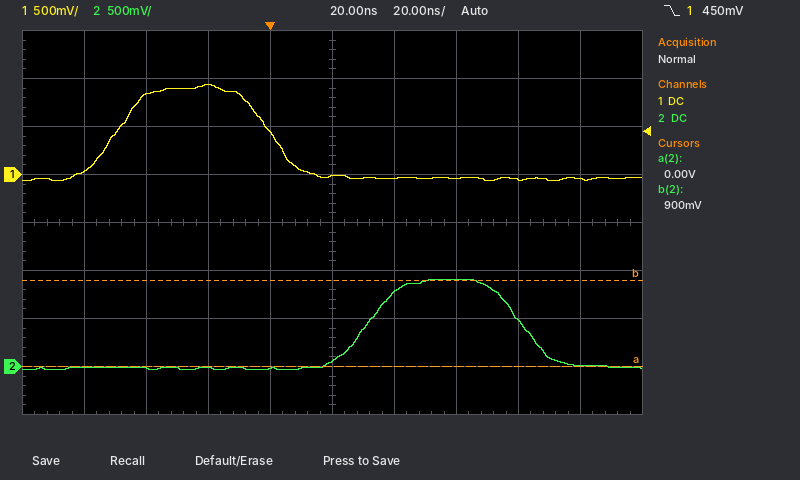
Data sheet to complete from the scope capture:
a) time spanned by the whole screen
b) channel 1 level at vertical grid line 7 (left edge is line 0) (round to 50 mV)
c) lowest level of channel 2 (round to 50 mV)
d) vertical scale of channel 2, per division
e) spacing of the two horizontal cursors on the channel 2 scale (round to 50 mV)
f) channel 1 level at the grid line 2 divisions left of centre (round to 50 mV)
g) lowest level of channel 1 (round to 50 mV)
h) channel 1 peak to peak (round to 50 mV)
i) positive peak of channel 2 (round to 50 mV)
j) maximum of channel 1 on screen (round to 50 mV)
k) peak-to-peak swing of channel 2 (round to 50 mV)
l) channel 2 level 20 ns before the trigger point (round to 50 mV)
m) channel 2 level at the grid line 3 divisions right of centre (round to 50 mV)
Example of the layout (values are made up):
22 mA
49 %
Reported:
200 ns
-50 mV
-50 mV
500 mV
900 mV
950 mV
-50 mV
1.00 V
900 mV
950 mV
950 mV
0 mV
500 mV
